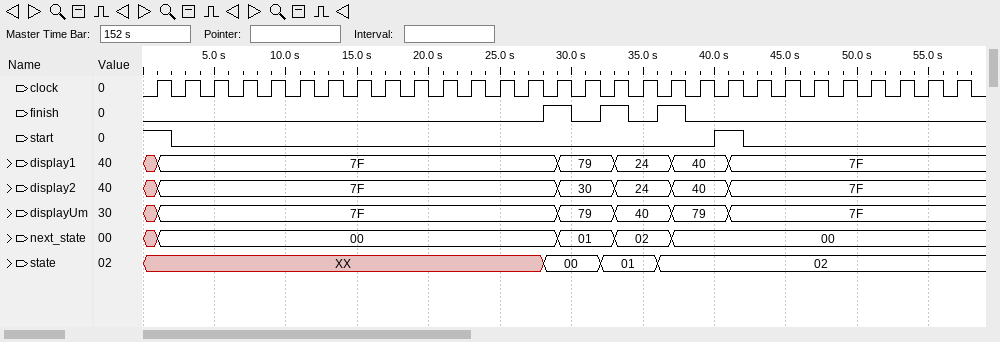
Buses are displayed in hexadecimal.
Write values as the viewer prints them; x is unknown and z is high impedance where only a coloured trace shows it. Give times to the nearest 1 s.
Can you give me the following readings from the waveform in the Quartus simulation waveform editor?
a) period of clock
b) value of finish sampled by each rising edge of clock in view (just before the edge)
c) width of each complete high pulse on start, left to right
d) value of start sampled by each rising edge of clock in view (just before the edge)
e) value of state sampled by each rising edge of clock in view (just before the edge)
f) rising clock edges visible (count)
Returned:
2 s
0 0 0 0 0 0 0 0 0 0 0 0 0 0 1 0 1 0 1 0 0 0 0 0 0 0 0 0 0
2 s
1 0 0 0 0 0 0 0 0 0 0 0 0 0 0 0 0 0 0 0 1 0 0 0 0 0 0 0 0
XX, XX, XX, XX, XX, XX, XX, XX, XX, XX, XX, XX, XX, XX, 00, 00, 01, 01, 02, 02, 02, 02, 02, 02, 02, 02, 02, 02, 02
29
